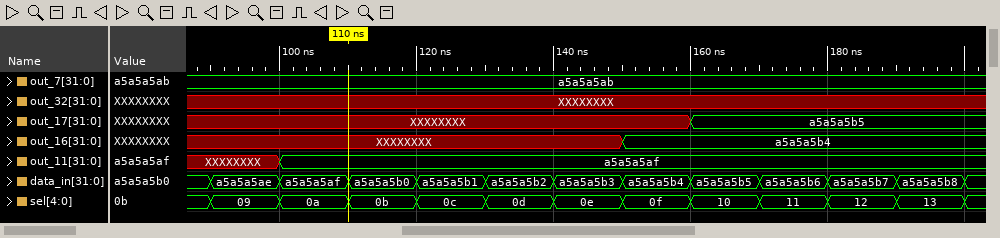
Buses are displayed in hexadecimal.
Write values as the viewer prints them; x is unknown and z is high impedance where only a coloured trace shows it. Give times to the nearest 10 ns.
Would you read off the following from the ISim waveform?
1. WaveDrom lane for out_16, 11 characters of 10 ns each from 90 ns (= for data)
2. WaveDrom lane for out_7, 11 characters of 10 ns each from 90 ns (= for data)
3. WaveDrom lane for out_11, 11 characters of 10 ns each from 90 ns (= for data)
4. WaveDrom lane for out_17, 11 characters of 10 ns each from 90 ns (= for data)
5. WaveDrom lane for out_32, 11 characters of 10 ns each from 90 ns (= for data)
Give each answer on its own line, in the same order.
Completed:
{name: 'out_16', wave: 'x.....=....', data: 'a5a5a5b4'}
{name: 'out_7', wave: '=..........', data: 'a5a5a5ab'}
{name: 'out_11', wave: 'x=.........', data: 'a5a5a5af'}
{name: 'out_17', wave: 'x......=...', data: 'a5a5a5b5'}
{name: 'out_32', wave: 'x..........'}
